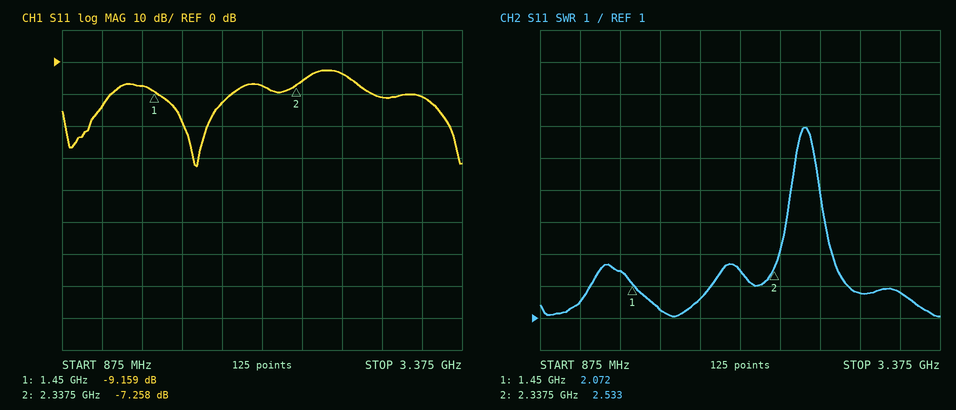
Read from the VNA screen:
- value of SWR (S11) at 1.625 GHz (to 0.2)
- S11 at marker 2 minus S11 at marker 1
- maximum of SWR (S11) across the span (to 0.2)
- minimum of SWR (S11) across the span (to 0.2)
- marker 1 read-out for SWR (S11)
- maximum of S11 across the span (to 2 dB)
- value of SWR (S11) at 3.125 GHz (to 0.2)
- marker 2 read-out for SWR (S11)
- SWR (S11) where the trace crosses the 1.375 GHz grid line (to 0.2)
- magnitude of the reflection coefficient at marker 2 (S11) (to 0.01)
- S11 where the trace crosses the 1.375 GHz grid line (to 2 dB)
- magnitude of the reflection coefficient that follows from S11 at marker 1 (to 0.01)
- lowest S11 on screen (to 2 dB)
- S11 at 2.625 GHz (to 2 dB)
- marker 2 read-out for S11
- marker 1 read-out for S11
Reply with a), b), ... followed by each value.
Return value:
a) 1.2
b) 1.901 dB
c) 7.0
d) 1.0
e) 2.072
f) -2 dB
g) 1.8
h) 2.533
i) 2.4
j) 0.43
k) -8 dB
l) 0.35
m) -32 dB
n) -4 dB
o) -7.258 dB
p) -9.159 dB
